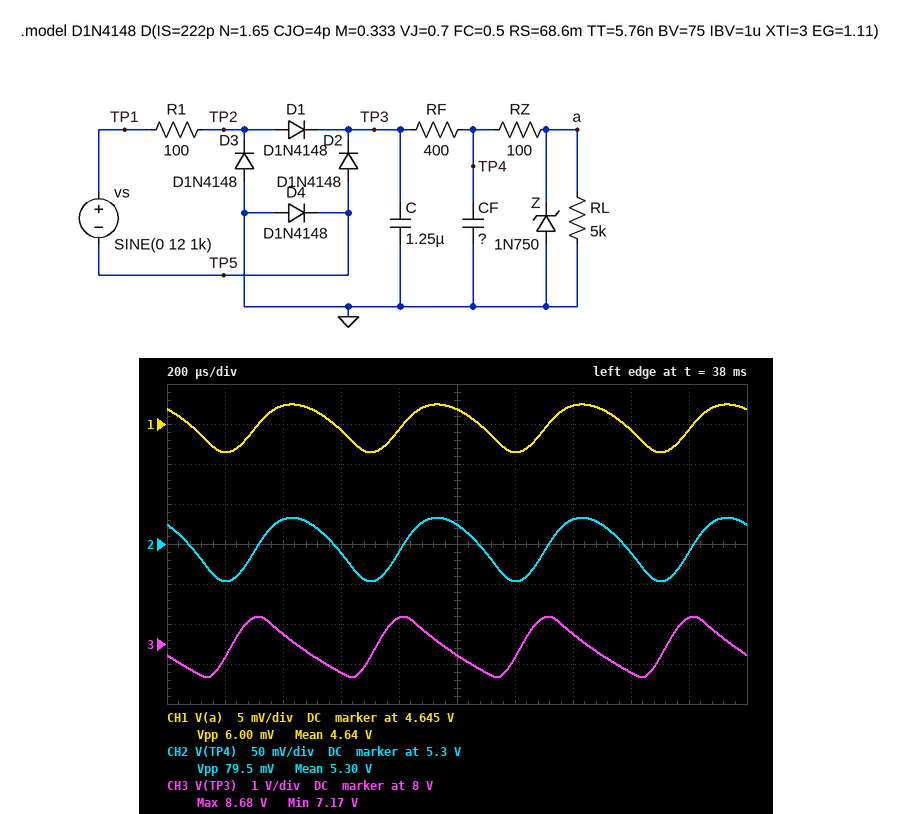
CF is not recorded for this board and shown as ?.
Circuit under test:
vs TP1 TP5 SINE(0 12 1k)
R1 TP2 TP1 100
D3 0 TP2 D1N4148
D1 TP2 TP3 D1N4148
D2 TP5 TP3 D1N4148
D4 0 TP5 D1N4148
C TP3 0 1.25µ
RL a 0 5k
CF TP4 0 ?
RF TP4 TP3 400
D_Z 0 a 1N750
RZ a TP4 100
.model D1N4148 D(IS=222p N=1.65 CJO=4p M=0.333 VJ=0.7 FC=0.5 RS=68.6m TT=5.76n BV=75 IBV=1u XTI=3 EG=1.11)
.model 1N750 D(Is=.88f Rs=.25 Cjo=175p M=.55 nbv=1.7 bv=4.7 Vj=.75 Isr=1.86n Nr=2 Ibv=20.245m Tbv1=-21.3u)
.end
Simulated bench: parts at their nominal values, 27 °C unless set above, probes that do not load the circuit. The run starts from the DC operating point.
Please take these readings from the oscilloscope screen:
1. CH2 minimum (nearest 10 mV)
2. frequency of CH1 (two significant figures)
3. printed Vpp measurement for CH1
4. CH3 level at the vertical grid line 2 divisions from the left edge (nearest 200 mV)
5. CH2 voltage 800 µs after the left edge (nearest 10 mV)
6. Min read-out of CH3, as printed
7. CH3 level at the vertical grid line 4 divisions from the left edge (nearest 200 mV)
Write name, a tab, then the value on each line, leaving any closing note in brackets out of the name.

CH2 minimum	5.25 V
frequency of CH1	2.0 kHz
printed Vpp measurement for CH1	6.00 mV
CH3 level at the vertical grid line 2 divisions from the left edge	8.2 V
CH2 voltage 800 µs after the left edge	5.29 V
Min read-out of CH3, as printed	7.17 V
CH3 level at the vertical grid line 4 divisions from the left edge	8.6 V
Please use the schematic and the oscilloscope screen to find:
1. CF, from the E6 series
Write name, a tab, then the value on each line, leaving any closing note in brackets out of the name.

CF, from the E6 series	3.3 µF
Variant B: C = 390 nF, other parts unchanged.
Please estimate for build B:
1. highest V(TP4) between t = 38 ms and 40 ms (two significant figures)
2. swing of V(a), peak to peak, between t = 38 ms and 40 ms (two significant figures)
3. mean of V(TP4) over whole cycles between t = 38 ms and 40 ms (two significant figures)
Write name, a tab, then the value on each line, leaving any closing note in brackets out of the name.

highest V(TP4) between t = 38 ms and 40 ms	5.3 V
swing of V(a), peak to peak, between t = 38 ms and 40 ms	17 mV
mean of V(TP4) over whole cycles between t = 38 ms and 40 ms	5.2 V
